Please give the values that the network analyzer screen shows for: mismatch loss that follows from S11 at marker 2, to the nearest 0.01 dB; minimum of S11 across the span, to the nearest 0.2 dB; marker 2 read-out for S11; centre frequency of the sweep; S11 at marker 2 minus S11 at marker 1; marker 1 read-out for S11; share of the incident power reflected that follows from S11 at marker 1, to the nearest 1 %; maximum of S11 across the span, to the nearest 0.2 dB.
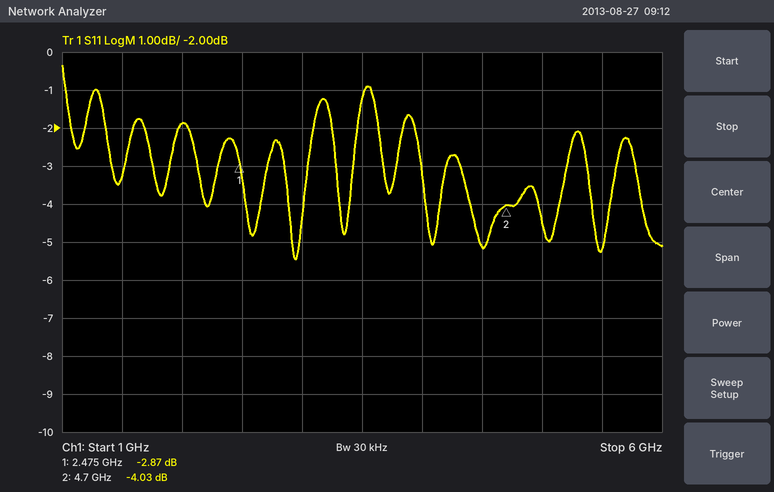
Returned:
2.19 dB
-5.4 dB
-4.03 dB
3.5 GHz
-1.16 dB
-2.87 dB
52 %
-0.4 dB
